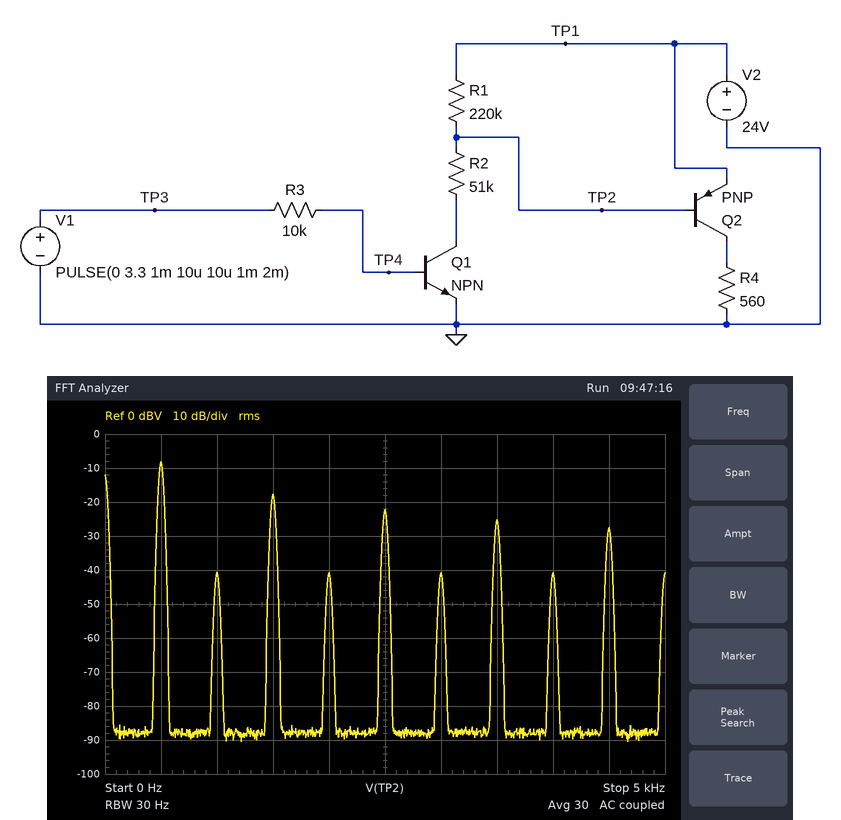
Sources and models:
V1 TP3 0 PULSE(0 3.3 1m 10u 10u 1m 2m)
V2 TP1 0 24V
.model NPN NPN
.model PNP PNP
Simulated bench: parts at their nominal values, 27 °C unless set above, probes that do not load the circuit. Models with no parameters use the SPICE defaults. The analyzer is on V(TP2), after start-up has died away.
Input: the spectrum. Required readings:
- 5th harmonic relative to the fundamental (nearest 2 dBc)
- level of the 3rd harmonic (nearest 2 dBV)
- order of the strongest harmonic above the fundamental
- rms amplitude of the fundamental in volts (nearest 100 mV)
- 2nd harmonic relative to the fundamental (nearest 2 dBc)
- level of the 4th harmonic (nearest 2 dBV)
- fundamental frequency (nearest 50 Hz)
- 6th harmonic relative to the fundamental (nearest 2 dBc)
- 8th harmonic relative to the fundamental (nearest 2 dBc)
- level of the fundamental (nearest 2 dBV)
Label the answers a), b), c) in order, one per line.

a) -14 dBc
b) -18 dBV
c) 3
d) 400 mV
e) -32 dBc
f) -40 dBV
g) 500 Hz
h) -32 dBc
i) -32 dBc
j) -8 dBV
